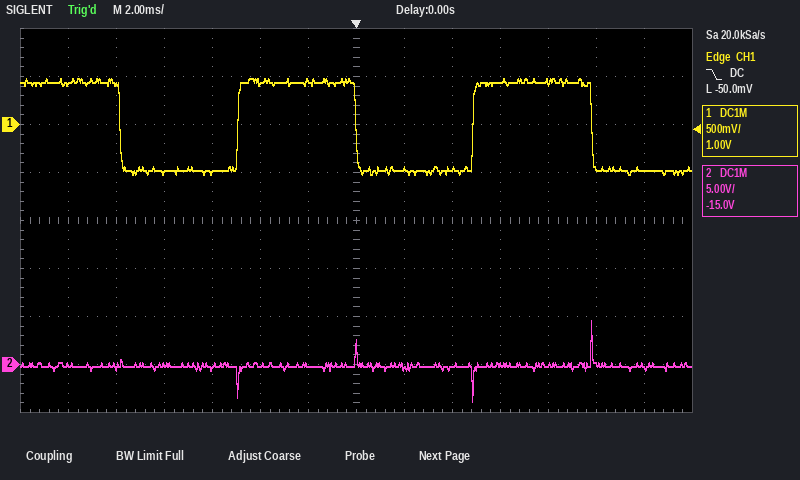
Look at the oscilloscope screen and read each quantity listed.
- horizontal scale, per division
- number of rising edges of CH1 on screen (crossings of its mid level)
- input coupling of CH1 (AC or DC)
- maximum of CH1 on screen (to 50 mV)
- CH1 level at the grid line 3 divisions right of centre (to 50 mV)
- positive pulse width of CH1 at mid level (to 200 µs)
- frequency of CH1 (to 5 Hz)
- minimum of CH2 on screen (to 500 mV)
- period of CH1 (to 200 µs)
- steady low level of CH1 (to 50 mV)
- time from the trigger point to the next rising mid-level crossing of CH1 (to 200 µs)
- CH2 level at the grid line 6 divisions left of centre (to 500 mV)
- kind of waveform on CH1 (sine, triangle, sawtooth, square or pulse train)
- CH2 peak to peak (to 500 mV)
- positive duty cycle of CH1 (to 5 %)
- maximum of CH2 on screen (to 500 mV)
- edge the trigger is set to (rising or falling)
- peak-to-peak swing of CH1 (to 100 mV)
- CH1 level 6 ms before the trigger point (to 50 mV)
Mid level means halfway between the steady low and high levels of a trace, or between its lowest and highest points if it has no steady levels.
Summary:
2 ms
2
DC
500 mV
450 mV
5.0 ms
100 Hz
-4.0 V
9.8 ms
-500 mV
4.8 ms
0.0 V
square
8.5 V
50 %
4.5 V
falling
1.00 V
-500 mV
